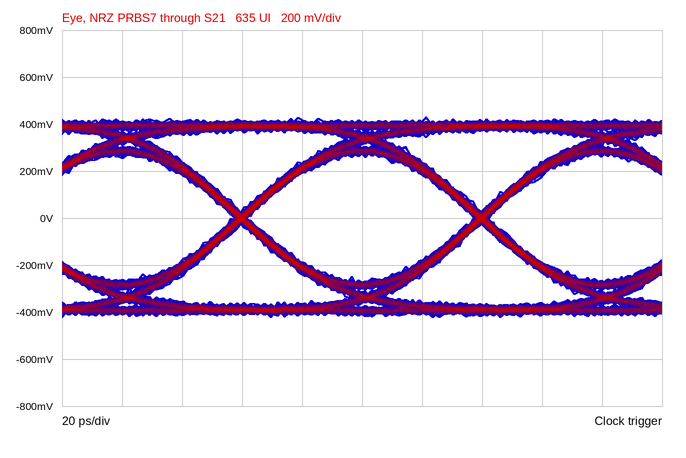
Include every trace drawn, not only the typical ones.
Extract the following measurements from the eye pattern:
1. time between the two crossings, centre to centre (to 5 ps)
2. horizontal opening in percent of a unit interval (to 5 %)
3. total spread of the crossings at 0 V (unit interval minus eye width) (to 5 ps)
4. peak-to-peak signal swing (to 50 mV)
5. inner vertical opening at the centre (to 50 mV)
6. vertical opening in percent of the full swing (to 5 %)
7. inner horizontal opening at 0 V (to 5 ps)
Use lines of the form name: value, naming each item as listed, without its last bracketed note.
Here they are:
time between the two crossings, centre to centre: 80 ps
horizontal opening in percent of a unit interval: 95 %
total spread of the crossings at 0 V (unit interval minus eye width): 5 ps
peak-to-peak signal swing: 850 mV
inner vertical opening at the centre: 550 mV
vertical opening in percent of the full swing: 65 %
inner horizontal opening at 0 V: 75 ps
